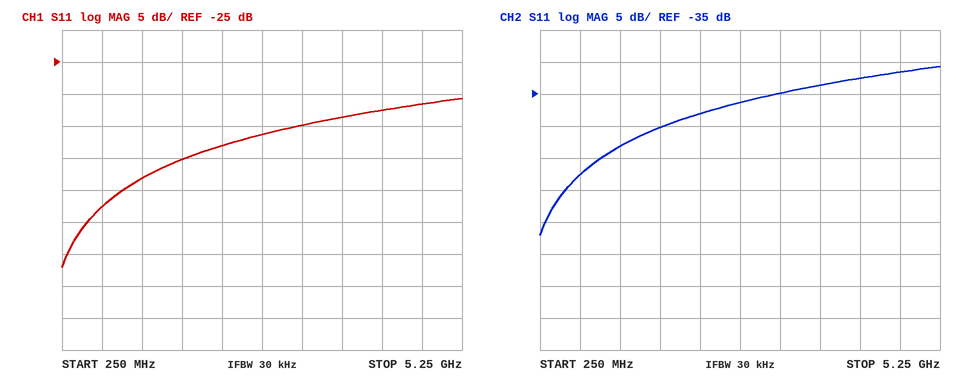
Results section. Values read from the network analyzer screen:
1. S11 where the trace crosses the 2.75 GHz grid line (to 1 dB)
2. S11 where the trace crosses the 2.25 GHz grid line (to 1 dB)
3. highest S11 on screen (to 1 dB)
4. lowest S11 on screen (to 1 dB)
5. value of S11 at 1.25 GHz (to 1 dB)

-36 dB
-38 dB
-31 dB
-57 dB
-43 dB
